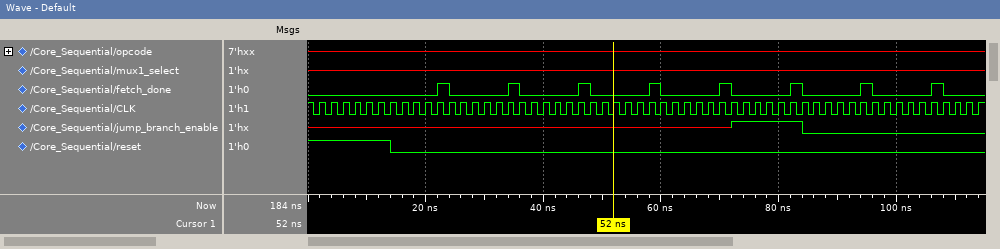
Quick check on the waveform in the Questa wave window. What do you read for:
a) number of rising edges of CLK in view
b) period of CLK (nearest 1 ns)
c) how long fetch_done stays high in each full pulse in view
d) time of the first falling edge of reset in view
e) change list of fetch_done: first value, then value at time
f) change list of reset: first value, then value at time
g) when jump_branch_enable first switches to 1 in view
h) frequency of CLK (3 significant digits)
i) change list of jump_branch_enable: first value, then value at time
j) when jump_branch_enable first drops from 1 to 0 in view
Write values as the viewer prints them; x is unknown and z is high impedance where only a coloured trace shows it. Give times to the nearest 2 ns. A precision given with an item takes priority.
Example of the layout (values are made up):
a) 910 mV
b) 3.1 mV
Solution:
a) 57
b) 2 ns
c) 2 ns, 2 ns, 2 ns, 2 ns, 2 ns, 2 ns, 2 ns, 2 ns
d) 14 ns
e) 0, 1 at 22 ns, 0 at 24 ns, 1 at 34 ns, 0 at 36 ns, 1 at 46 ns, 0 at 48 ns, 1 at 58 ns, 0 at 60 ns, 1 at 70 ns, 0 at 72 ns, 1 at 82 ns, 0 at 84 ns, 1 at 94 ns, 0 at 96 ns, 1 at 106 ns, 0 at 108 ns
f) 1, 0 at 14 ns
g) 72 ns
h) 500 MHz
i) x, 1 at 72 ns, 0 at 84 ns
j) 84 ns
